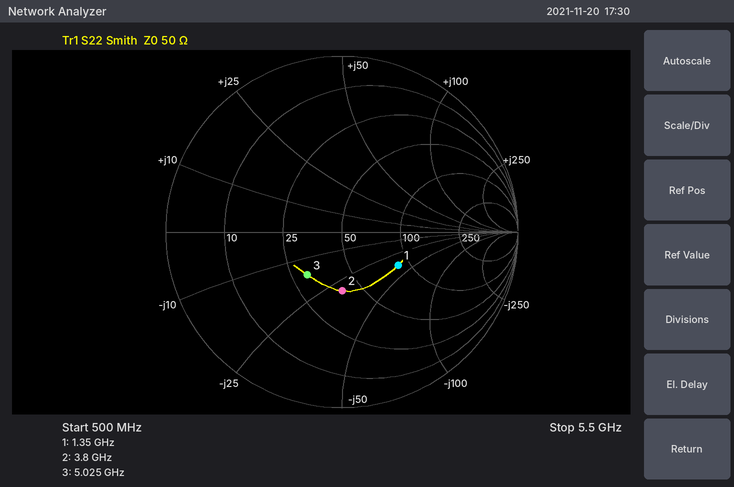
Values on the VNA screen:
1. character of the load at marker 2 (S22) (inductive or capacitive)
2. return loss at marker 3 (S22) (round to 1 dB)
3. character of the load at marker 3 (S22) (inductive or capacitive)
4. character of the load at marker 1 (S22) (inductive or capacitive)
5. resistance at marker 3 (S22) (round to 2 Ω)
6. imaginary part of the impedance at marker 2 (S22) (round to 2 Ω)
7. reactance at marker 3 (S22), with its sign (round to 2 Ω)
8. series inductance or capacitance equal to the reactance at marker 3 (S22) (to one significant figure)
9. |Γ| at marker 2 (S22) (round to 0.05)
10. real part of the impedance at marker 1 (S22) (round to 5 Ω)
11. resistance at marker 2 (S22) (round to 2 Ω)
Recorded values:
capacitive
10 dB
capacitive
capacitive
30 Ω
-30 Ω
-16 Ω
2 pF
0.35
85 Ω
40 Ω
